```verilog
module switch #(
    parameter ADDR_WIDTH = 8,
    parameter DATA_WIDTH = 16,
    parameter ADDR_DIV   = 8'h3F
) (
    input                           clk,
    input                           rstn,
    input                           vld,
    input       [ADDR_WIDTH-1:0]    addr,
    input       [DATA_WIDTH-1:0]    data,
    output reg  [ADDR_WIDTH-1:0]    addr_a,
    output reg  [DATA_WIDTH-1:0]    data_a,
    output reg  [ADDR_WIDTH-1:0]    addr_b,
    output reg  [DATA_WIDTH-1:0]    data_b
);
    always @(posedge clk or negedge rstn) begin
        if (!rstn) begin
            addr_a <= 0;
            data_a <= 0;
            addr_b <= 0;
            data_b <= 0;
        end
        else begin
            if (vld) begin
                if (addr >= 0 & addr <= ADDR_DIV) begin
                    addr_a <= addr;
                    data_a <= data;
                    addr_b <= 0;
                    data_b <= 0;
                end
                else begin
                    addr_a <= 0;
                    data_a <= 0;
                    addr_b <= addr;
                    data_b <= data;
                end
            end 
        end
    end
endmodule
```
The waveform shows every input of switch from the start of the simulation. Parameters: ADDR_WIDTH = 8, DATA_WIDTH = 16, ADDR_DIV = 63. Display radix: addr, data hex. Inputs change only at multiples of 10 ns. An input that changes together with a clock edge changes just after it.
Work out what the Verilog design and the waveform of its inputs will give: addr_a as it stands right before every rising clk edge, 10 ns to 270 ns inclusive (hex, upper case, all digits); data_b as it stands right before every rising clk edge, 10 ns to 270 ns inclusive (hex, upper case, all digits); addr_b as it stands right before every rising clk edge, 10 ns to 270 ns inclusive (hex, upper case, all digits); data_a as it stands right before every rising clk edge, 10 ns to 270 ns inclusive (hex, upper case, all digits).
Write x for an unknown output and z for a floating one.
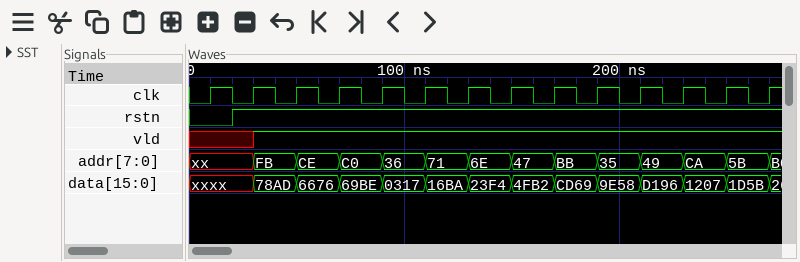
00, 00, 00, 00, 00, 00, 36, 00, 00, 00, 00, 35, 00, 00
0000, 0000, 0000, 78AD, 6676, 69BE, 0000, 16BA, 23F4, 4FB2, CD69, 0000, D196, 1207
00, 00, 00, FB, CE, C0, 00, 71, 6E, 47, BB, 00, 49, CA
0000, 0000, 0000, 0000, 0000, 0000, 0317, 0000, 0000, 0000, 0000, 9E58, 0000, 0000
